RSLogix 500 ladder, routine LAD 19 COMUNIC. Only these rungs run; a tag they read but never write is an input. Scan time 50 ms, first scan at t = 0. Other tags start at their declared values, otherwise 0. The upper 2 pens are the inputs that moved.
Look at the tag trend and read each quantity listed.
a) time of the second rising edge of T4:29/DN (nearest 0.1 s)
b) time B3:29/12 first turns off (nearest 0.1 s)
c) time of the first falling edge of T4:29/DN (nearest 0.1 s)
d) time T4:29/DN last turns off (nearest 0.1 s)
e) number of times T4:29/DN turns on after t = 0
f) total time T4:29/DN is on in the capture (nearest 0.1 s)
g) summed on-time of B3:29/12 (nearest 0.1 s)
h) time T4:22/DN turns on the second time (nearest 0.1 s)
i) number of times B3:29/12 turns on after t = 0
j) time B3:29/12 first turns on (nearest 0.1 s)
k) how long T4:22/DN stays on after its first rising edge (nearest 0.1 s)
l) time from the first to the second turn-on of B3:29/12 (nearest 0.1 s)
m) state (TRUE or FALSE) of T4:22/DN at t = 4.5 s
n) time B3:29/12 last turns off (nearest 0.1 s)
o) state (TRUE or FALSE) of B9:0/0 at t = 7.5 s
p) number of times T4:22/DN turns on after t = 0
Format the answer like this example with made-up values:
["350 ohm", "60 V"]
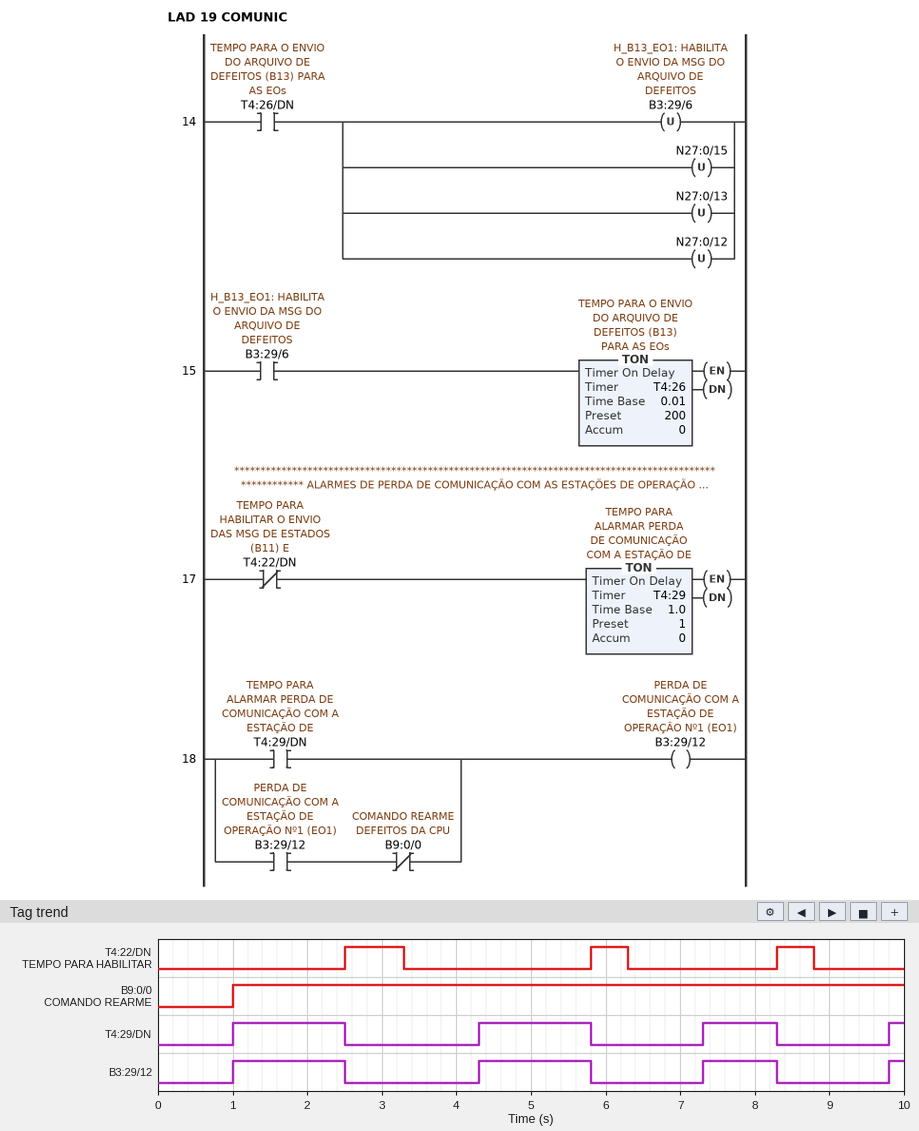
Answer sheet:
["4.3 s", "2.5 s", "2.5 s", "8.3 s", "4", "4.2 s", "4.2 s", "5.8 s", "4", "1.0 s", "0.8 s", "3.3 s", "FALSE", "8.3 s", "TRUE", "3"]
